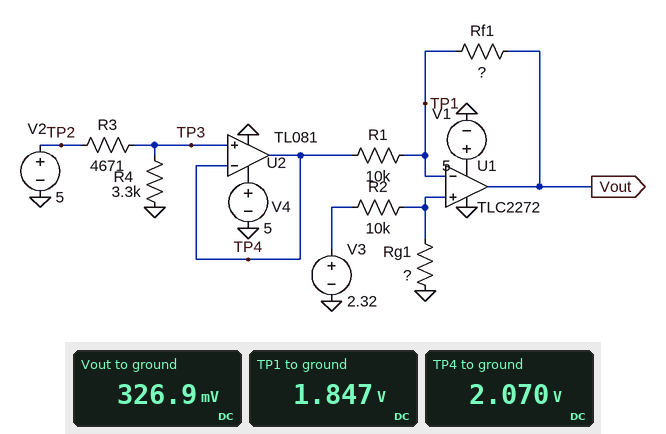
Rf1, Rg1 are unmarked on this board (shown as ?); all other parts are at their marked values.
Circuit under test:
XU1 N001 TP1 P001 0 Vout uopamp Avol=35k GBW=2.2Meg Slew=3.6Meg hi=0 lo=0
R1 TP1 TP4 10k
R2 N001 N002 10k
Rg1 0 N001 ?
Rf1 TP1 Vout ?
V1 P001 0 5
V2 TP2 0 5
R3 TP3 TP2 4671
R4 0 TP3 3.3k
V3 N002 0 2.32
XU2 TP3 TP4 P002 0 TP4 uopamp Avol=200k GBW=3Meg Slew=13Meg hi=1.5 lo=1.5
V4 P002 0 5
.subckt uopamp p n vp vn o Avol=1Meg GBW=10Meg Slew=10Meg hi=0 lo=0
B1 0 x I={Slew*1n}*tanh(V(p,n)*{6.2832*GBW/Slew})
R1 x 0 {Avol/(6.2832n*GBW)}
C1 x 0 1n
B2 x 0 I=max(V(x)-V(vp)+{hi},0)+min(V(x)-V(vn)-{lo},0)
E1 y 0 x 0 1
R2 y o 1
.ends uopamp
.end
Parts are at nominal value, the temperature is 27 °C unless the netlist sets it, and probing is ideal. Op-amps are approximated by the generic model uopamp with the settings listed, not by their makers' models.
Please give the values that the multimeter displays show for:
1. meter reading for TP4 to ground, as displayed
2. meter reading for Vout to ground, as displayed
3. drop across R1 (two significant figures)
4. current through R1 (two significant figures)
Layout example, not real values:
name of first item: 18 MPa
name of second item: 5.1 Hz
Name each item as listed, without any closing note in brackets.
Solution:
meter reading for TP4 to ground, as displayed: 2.070 V
meter reading for Vout to ground, as displayed: 326.9 mV
drop across R1: 220 mV
current through R1: 22 µA
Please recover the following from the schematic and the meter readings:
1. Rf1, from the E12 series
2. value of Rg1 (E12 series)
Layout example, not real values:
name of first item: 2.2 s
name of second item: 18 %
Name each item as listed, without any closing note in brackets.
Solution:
Rf1, from the E12 series: 68 kΩ
value of Rg1: 39 kΩ
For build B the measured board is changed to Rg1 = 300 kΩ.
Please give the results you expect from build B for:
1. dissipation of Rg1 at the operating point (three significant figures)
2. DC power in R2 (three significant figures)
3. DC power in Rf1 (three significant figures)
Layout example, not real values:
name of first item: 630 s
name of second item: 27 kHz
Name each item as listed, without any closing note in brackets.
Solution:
dissipation of Rg1 at the operating point: 16.8 µW
DC power in R2: 560 nW
DC power in Rf1: 20.8 µW
